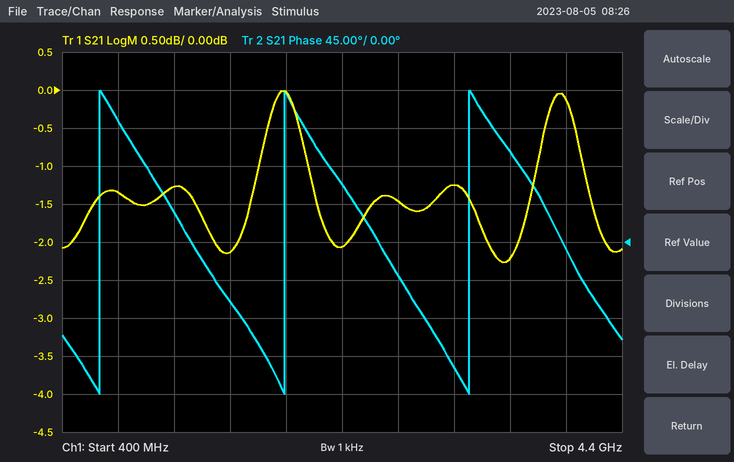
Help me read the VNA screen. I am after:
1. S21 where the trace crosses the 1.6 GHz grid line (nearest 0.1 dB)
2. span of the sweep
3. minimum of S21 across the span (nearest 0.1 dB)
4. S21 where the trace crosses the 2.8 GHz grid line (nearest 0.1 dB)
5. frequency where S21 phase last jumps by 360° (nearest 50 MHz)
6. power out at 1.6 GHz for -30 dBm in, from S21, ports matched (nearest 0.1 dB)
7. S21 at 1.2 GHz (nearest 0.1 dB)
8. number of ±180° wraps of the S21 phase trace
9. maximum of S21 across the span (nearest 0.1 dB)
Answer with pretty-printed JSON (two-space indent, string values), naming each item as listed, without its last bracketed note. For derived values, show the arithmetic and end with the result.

{
  "S21 where the trace crosses the 1.6 GHz grid line": "-2.1 dB",
  "span of the sweep": "4 GHz",
  "minimum of S21 across the span": "-2.3 dB",
  "S21 where the trace crosses the 2.8 GHz grid line": "-1.5 dB",
  "frequency where S21 phase last jumps by 360°": "3.30 GHz",
  "power out at 1.6 GHz for -30 dBm in, from S21, ports matched": "-30 dBm + (-2.1 dB) = -32.1 dBm",
  "S21 at 1.2 GHz": "-1.3 dB",
  "number of ±180° wraps of the S21 phase trace": "3",
  "maximum of S21 across the span": "0.0 dB"
}
